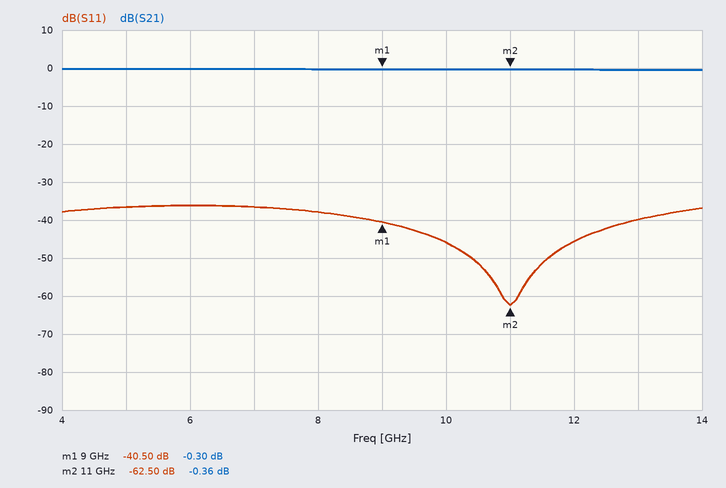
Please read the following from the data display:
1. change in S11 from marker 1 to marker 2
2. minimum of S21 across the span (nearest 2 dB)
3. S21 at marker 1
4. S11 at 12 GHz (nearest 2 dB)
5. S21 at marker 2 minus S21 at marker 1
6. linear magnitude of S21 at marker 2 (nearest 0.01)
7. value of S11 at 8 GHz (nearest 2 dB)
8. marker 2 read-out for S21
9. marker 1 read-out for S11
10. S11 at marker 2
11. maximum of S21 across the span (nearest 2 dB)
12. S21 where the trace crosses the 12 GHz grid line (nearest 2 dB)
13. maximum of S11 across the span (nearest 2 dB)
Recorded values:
-22.00 dB
0 dB
-0.30 dB
-46 dB
-0.06 dB
0.96
-38 dB
-0.36 dB
-40.50 dB
-62.50 dB
0 dB
0 dB
-36 dB
